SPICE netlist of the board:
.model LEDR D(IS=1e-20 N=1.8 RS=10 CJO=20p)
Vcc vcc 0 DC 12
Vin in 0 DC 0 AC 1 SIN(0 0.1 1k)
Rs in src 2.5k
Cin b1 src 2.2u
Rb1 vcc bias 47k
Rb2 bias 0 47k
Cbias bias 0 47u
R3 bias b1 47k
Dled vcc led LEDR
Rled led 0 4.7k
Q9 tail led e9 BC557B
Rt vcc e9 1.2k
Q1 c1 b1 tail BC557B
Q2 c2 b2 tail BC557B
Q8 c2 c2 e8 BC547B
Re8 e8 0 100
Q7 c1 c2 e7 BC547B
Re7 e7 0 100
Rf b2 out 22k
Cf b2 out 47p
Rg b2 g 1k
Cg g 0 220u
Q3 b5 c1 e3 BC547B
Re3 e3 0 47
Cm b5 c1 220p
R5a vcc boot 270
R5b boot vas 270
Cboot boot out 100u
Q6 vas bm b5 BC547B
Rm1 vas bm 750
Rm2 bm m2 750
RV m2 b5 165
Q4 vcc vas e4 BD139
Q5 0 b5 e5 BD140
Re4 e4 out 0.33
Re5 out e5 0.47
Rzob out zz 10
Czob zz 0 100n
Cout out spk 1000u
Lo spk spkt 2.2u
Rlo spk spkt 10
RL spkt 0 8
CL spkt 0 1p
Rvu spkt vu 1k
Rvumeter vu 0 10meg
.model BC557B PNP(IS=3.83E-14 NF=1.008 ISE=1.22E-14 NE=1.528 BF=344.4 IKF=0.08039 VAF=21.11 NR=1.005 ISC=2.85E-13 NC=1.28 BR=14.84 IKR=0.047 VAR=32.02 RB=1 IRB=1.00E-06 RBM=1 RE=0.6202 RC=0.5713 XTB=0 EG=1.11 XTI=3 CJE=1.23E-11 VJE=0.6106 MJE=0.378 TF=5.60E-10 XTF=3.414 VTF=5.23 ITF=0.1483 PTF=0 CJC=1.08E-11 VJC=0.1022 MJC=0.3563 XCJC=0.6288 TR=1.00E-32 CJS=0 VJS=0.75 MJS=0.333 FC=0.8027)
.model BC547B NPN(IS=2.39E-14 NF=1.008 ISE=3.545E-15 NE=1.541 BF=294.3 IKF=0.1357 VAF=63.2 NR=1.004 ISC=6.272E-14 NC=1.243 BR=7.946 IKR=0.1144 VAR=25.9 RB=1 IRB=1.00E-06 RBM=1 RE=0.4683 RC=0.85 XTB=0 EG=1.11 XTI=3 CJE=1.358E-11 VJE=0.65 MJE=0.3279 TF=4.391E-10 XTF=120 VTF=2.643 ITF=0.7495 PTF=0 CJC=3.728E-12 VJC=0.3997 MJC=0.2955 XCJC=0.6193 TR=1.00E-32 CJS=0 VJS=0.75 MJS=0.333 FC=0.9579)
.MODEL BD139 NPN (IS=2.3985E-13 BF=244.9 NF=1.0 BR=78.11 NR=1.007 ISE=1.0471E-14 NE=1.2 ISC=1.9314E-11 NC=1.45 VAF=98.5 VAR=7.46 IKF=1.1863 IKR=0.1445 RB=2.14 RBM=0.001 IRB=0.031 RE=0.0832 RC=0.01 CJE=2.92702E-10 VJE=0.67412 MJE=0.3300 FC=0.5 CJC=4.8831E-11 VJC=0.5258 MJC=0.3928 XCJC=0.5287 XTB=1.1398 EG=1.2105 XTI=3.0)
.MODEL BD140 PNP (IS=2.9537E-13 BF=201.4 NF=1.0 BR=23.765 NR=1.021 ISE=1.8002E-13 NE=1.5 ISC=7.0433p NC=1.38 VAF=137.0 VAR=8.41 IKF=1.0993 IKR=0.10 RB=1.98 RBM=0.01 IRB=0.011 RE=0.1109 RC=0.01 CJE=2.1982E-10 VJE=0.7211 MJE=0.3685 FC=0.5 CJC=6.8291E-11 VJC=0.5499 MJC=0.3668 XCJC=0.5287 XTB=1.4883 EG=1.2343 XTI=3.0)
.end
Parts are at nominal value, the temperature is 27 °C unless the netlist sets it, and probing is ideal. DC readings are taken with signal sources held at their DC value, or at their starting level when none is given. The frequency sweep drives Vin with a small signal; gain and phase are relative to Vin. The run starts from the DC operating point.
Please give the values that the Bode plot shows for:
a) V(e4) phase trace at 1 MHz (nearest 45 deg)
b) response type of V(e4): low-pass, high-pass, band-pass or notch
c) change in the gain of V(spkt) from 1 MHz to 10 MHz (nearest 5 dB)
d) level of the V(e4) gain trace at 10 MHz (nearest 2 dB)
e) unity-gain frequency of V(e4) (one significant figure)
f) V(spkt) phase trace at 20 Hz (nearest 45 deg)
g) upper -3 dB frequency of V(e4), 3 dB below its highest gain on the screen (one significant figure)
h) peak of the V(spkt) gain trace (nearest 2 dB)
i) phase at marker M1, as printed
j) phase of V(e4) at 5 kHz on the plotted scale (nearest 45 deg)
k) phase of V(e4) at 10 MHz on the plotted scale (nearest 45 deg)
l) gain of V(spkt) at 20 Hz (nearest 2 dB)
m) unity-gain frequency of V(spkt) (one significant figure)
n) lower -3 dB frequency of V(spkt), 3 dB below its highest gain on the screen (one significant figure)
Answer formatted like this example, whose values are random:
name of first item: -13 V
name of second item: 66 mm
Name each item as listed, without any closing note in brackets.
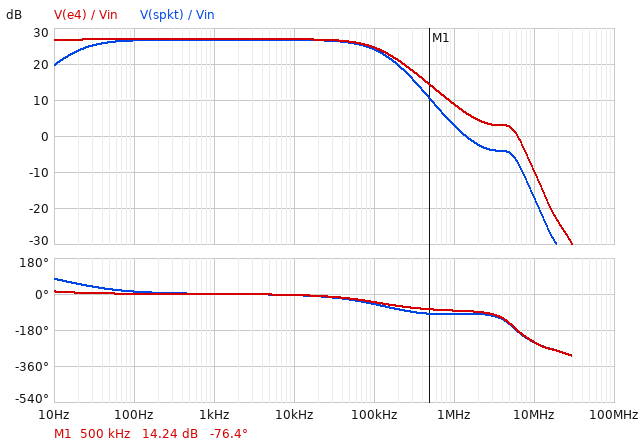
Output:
V(e4) phase trace at 1 MHz: -90 deg
response type of V(e4): low-pass, high-pass, band-pass or notch: low-pass
change in the gain of V(spkt) from 1 MHz to 10 MHz: -20 dB
level of the V(e4) gain trace at 10 MHz: -10 dB
unity-gain frequency of V(e4): 6 MHz
V(spkt) phase trace at 20 Hz: 45 deg
upper -3 dB frequency of V(e4), 3 dB below its highest gain on the screen: 100 kHz
peak of the V(spkt) gain trace: 26 dB
phase at marker M1, as printed: -76.4 deg
phase of V(e4) at 5 kHz on the plotted scale: 0 deg
phase of V(e4) at 10 MHz on the plotted scale: -225 deg
gain of V(spkt) at 20 Hz: 24 dB
unity-gain frequency of V(spkt): 1 MHz
lower -3 dB frequency of V(spkt), 3 dB below its highest gain on the screen: 20 Hz
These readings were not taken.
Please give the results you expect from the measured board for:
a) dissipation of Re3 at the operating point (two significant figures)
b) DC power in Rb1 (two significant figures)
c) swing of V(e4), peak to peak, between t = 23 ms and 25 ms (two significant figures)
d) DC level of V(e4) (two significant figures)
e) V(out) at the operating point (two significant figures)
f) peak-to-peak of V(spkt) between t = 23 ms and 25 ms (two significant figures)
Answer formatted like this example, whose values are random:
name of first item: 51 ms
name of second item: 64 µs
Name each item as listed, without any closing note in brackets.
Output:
dissipation of Re3 at the operating point: 4.5 mW
DC power in Rb1: 760 µW
swing of V(e4), peak to peak, between t = 23 ms and 25 ms: 4.4 V
DC level of V(e4): 6.1 V
V(out) at the operating point: 6.1 V
peak-to-peak of V(spkt) between t = 23 ms and 25 ms: 4.3 V
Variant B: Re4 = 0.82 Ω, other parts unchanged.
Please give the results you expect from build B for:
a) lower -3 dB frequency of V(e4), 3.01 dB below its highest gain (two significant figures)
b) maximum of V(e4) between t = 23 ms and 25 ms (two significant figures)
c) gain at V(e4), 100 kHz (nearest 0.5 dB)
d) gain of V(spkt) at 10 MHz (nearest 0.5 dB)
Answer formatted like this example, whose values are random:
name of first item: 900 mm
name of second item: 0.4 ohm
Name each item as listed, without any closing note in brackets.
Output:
lower -3 dB frequency of V(e4), 3.01 dB below its highest gain: 2.0 Hz
maximum of V(e4) between t = 23 ms and 25 ms: 8.5 V
gain at V(e4), 100 kHz: 25.0 dB
gain of V(spkt) at 10 MHz: -17.5 dB
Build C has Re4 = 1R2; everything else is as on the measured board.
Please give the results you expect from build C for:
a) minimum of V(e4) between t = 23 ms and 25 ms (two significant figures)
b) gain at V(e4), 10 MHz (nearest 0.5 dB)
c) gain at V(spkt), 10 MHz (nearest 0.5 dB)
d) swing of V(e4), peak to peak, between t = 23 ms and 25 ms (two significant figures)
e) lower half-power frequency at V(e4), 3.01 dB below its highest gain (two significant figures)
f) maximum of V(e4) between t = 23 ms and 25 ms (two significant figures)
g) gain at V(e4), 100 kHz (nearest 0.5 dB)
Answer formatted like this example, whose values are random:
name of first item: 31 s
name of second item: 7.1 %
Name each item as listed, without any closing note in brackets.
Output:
minimum of V(e4) between t = 23 ms and 25 ms: 3.9 V
gain at V(e4), 10 MHz: -10.0 dB
gain at V(spkt), 10 MHz: -17.5 dB
swing of V(e4), peak to peak, between t = 23 ms and 25 ms: 4.7 V
lower half-power frequency at V(e4), 3.01 dB below its highest gain: 2.1 Hz
maximum of V(e4) between t = 23 ms and 25 ms: 8.6 V
gain at V(e4), 100 kHz: 25.0 dB
